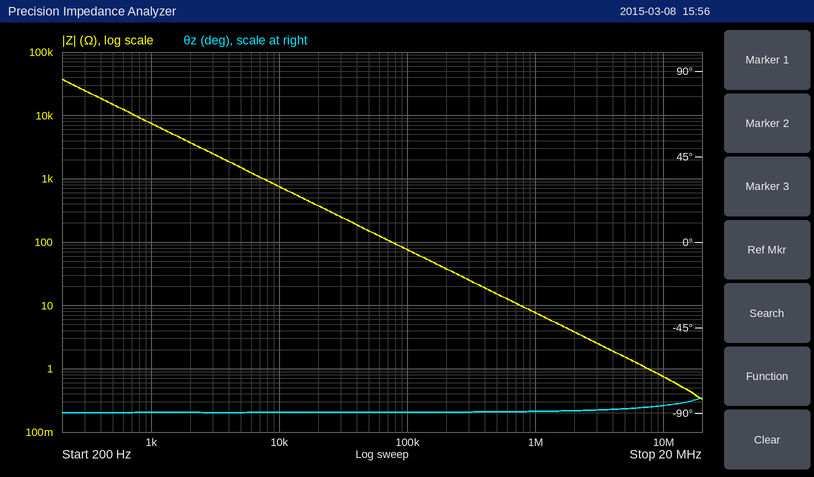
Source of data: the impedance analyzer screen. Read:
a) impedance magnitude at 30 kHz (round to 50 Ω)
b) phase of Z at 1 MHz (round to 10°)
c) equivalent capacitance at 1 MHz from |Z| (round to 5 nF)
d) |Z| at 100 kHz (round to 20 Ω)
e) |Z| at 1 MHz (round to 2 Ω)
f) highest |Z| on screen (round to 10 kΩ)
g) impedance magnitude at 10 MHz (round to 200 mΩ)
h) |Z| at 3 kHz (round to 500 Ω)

250 Ω
-90°
20 nF
80 Ω
8 Ω
40 kΩ
800 mΩ
2.5 kΩ
